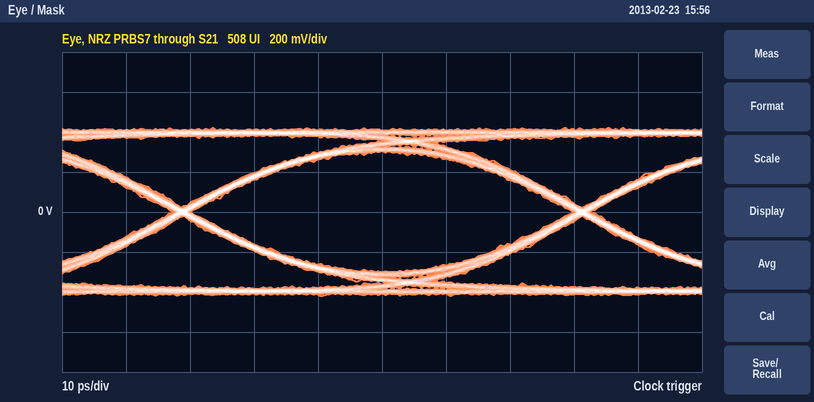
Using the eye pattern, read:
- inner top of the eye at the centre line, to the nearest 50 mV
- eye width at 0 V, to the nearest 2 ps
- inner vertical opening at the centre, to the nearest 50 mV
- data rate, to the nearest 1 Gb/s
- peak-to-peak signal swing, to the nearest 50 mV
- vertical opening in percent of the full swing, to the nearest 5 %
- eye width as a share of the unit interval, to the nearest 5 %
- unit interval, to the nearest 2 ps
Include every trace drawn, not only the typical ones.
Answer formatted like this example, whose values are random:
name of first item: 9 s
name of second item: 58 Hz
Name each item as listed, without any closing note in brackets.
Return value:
inner top of the eye at the centre line, to the nearest 50 mV: 300 mV
eye width at 0 V, to the nearest 2 ps: 60 ps
inner vertical opening at the centre, to the nearest 50 mV: 600 mV
data rate, to the nearest 1 Gb/s: 16 Gb/s
peak-to-peak signal swing, to the nearest 50 mV: 850 mV
vertical opening in percent of the full swing, to the nearest 5 %: 70 %
eye width as a share of the unit interval, to the nearest 5 %: 95 %
unit interval, to the nearest 2 ps: 62 ps
